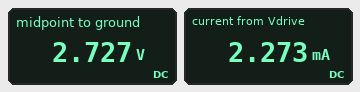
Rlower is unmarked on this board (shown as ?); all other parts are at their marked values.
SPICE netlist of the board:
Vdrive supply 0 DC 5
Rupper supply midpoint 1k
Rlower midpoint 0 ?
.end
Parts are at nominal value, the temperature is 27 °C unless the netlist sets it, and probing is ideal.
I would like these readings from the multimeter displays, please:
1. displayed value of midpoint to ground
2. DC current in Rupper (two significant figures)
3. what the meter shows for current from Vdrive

2.727 V
2.3 mA
2.273 mA
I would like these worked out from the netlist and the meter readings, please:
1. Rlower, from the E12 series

1.2 kΩ
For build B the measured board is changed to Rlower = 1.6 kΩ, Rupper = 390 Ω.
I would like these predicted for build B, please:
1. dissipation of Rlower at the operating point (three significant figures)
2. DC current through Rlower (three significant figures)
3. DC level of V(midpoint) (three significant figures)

10.1 mW
2.51 mA
4.02 V
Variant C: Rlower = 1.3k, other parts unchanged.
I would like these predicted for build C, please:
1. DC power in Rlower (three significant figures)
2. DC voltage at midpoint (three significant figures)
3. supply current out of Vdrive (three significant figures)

6.14 mW
2.83 V
2.17 mA
